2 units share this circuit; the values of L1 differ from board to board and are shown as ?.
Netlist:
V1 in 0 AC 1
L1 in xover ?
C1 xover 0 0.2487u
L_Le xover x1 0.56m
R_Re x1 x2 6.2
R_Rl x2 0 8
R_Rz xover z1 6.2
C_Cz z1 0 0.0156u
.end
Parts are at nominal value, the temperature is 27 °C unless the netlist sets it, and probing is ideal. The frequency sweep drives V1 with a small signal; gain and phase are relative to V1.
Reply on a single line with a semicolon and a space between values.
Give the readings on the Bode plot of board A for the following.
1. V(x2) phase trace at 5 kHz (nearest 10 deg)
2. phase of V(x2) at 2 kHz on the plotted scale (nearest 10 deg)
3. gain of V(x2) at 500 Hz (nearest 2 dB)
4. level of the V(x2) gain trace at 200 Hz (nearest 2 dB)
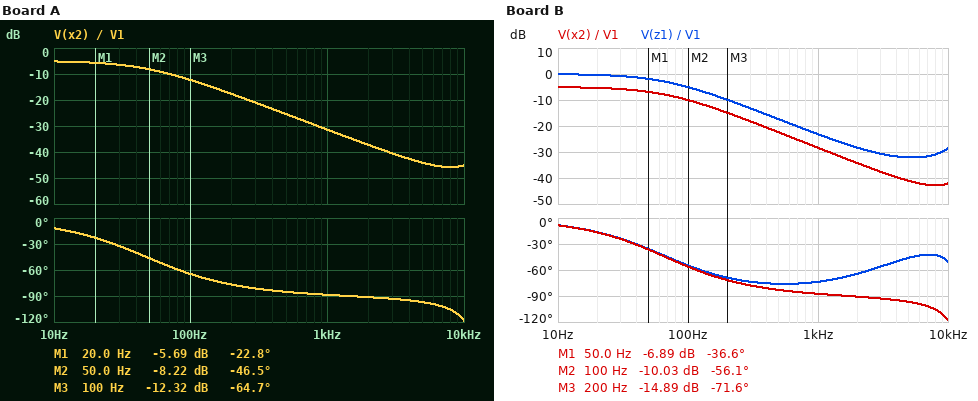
-100 deg; -90 deg; -26 dB; -18 dB
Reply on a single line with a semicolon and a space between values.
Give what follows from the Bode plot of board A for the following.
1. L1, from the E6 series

47 mH
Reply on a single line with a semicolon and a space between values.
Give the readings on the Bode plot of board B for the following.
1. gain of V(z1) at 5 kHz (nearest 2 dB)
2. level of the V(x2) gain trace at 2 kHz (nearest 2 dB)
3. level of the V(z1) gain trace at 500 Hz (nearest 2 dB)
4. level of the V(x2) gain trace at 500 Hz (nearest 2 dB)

-32 dB; -34 dB; -18 dB; -22 dB
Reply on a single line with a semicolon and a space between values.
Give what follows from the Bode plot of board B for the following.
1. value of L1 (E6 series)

33 mH
